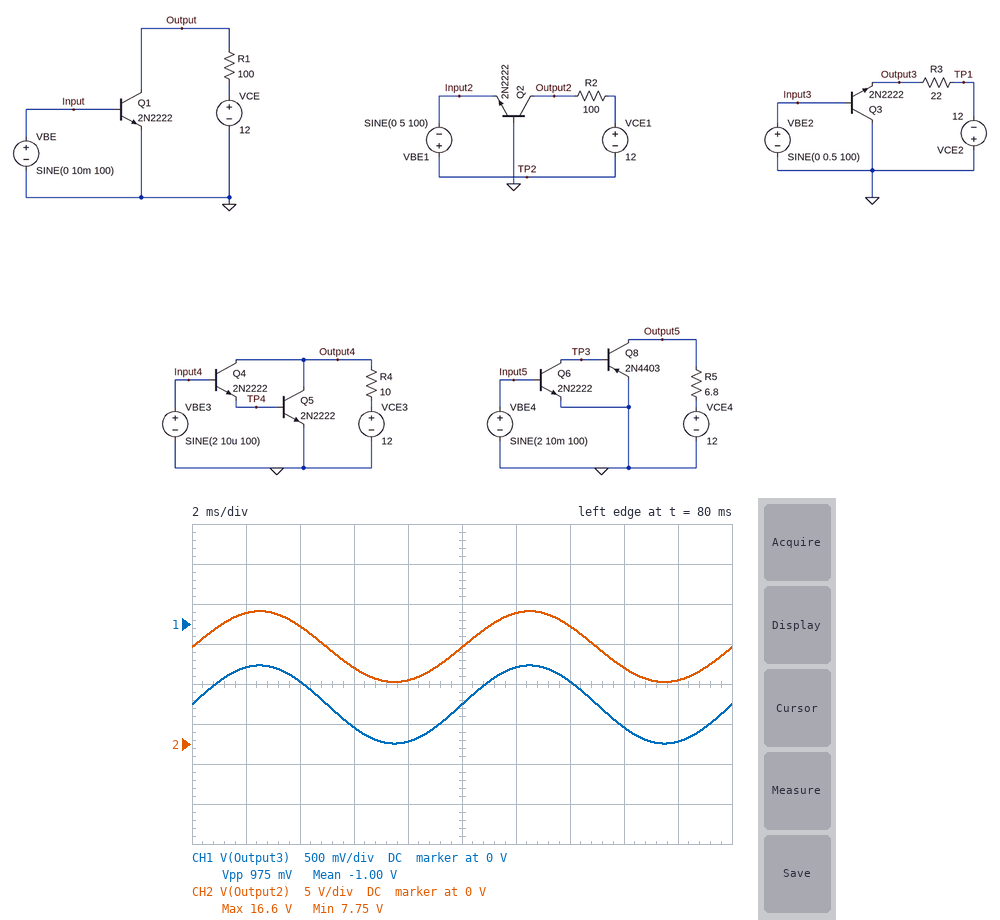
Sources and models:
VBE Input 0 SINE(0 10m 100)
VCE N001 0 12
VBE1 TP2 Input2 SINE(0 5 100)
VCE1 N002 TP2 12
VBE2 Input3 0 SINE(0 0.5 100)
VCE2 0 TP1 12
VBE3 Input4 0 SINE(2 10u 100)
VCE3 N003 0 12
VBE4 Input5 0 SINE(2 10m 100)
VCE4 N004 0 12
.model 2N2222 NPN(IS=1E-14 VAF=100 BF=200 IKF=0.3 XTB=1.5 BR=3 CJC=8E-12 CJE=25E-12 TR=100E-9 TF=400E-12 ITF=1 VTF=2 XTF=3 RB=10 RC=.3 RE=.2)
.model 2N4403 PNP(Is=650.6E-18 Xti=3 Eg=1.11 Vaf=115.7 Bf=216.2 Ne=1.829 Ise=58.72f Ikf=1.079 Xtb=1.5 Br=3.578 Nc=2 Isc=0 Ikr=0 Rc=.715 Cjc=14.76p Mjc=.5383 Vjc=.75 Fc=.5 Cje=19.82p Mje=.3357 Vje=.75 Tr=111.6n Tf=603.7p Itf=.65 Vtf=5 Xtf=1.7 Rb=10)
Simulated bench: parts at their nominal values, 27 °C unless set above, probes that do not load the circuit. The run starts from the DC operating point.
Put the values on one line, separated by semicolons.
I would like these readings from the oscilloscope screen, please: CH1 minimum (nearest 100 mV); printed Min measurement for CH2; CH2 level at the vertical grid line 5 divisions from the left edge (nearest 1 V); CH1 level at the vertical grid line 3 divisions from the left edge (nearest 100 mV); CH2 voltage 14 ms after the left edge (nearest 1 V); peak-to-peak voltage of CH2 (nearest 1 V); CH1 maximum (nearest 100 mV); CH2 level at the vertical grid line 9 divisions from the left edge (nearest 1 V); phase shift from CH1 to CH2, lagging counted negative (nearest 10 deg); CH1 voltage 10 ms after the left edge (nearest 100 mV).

-1.5 V; 7.75 V; 12 V; -1.3 V; 15 V; 9 V; -500 mV; 8 V; 0 deg; -1.0 V
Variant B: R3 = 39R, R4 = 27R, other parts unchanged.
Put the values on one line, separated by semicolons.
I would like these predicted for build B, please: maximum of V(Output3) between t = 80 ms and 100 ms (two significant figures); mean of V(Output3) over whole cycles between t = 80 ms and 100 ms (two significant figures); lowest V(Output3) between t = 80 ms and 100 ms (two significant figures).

-410 mV; -900 mV; -1.4 V
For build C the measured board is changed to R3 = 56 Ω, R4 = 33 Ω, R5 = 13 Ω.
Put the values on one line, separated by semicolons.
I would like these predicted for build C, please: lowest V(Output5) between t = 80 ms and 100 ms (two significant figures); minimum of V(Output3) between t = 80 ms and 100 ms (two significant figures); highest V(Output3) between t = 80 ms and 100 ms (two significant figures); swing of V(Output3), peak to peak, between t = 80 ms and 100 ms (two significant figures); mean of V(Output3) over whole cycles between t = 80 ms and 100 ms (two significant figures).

3.0 V; -1.4 V; -370 mV; 990 mV; -860 mV
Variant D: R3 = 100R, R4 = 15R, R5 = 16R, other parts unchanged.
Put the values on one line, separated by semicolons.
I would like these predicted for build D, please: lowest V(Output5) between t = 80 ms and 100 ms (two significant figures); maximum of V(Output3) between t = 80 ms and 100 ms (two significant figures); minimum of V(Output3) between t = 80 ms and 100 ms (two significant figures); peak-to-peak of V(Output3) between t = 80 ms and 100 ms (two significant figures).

2.7 V; -320 mV; -1.3 V; 990 mV
